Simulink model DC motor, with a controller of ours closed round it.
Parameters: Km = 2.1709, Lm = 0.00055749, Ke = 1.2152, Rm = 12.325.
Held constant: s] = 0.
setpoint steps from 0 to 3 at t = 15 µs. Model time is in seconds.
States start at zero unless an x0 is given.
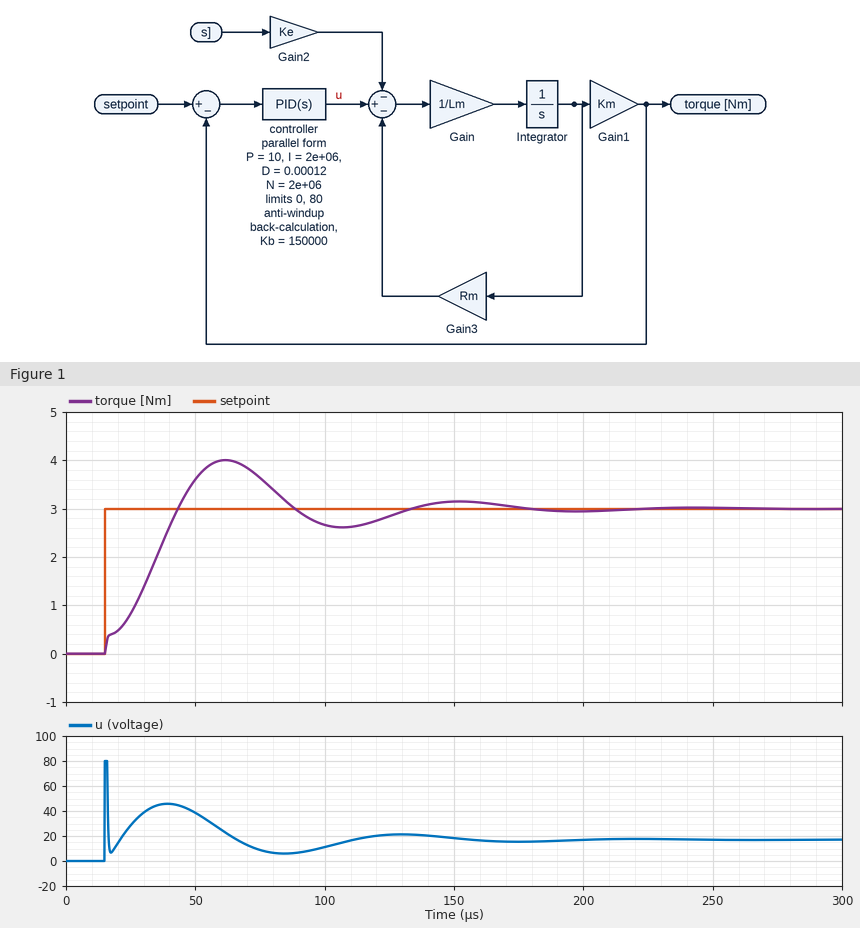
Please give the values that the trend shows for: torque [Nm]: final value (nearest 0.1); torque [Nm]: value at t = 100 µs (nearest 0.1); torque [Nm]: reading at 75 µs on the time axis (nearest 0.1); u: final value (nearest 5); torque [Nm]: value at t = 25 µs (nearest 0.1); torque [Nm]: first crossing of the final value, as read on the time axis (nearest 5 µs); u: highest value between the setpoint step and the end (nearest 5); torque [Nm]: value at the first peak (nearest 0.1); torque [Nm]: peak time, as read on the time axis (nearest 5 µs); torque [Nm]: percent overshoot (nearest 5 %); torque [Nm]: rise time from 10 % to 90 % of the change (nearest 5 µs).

3.0
2.7
3.6
15
0.8
45 µs
80
4.0
60 µs
35 %
25 µs
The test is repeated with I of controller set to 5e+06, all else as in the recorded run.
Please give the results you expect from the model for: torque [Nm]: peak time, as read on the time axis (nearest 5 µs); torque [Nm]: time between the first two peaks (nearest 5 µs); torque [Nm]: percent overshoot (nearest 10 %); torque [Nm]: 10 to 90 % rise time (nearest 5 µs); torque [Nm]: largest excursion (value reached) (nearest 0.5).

45 µs
60 µs
50 %
15 µs
4.5
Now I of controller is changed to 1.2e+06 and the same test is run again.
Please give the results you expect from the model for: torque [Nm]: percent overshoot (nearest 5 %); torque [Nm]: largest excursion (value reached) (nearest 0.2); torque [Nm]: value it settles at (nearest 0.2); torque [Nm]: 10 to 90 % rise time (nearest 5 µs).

25 %
3.8
3.0
35 µs
